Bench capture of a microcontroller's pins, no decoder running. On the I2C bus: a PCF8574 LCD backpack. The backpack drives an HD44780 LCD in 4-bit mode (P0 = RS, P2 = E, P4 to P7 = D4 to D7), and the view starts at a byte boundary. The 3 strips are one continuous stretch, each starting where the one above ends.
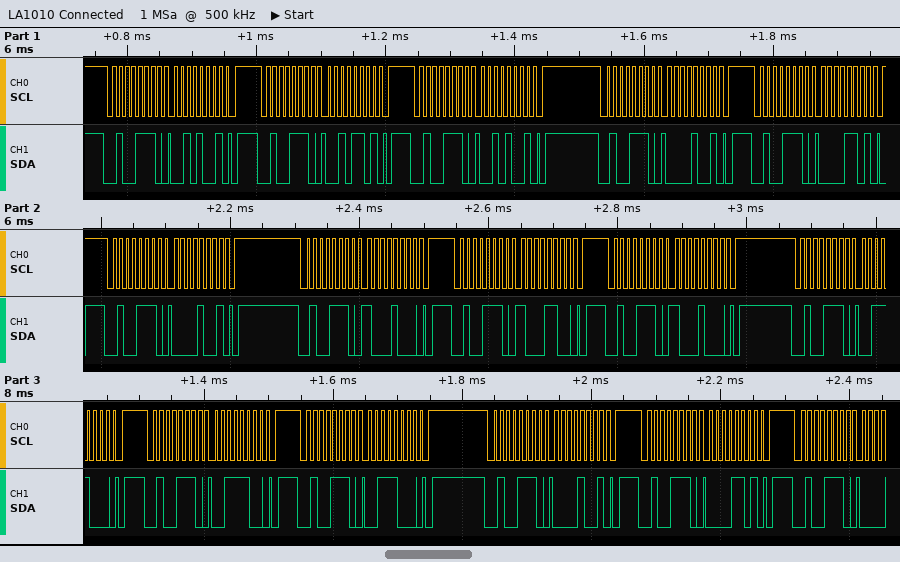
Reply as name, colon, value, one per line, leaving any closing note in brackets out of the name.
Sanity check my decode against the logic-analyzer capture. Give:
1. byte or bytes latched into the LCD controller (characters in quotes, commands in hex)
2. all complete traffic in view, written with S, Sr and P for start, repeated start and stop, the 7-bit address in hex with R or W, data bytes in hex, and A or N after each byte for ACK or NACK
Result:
byte or bytes latched into the LCD controller: ' ' 0x83
all complete traffic in view, written with S, Sr and P for start, repeated start and stop, the 7-bit address in hex with R or W, data bytes in hex, and A or N after each byte for ACK or NACK: S 27W A 29 A P S 27W A 2D A P S 27W A 29 A P S 27W A 09 A P S 27W A 0D A P S 27W A 09 A P S 27W A 88 A P S 27W A 8C A P S 27W A 88 A P S 27W A 38 A P S 27W A 3C A P S 27W A 38 A P S 27W A 09 A P S 27W A 0D A P S 27W A
